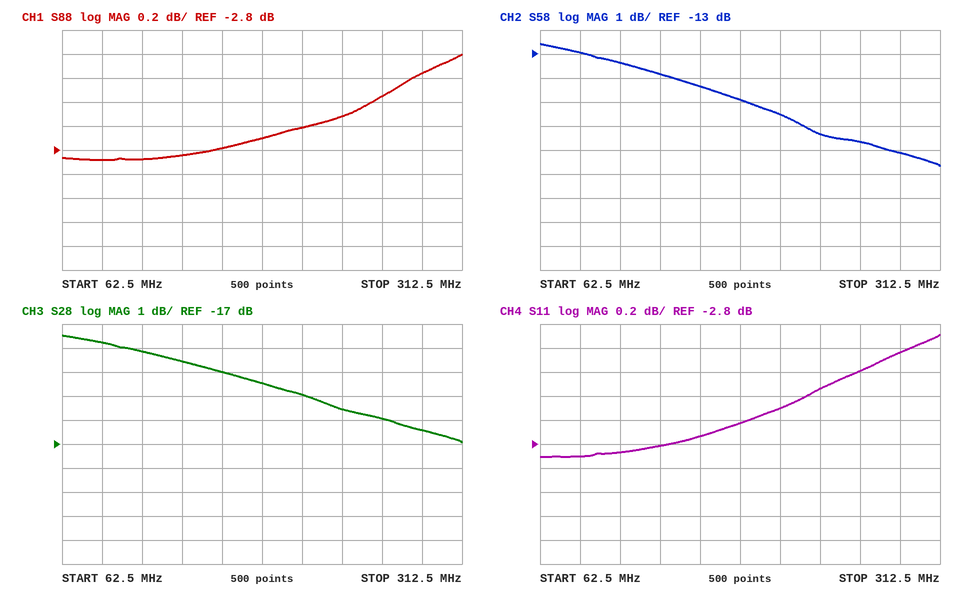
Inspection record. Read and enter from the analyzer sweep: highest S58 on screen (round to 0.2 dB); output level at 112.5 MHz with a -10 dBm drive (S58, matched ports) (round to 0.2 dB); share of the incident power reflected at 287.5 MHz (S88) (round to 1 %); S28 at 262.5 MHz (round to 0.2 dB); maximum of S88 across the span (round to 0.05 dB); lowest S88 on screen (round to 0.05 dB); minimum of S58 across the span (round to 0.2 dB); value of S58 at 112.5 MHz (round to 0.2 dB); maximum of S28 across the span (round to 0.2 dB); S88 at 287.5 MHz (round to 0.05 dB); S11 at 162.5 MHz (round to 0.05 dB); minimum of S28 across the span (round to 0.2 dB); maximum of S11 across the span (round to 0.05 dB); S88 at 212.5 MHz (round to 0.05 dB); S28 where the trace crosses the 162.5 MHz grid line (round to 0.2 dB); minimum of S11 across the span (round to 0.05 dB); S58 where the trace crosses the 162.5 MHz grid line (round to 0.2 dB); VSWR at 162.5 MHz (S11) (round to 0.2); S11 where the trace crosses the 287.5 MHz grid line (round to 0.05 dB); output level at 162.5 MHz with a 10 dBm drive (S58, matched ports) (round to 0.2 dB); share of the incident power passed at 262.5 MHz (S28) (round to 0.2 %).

-12.6 dB
-23.4 dBm
61 %
-16.0 dB
-2.00 dB
-2.90 dB
-17.6 dB
-13.4 dB
-12.4 dB
-2.15 dB
-2.75 dB
-17.0 dB
-1.90 dB
-2.60 dB
-14.0 dB
-2.90 dB
-14.4 dB
6.4
-2.05 dB
-4.4 dBm
2.6 %
